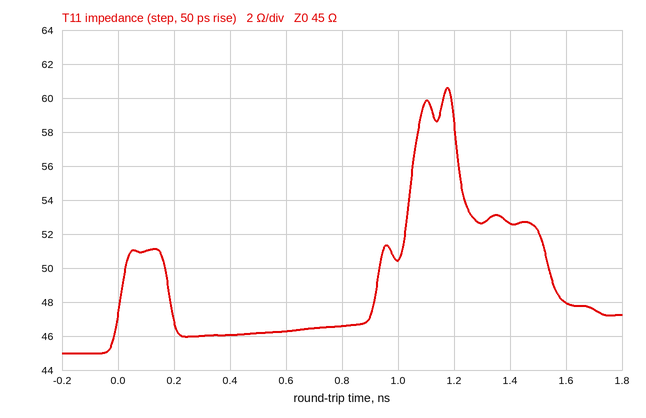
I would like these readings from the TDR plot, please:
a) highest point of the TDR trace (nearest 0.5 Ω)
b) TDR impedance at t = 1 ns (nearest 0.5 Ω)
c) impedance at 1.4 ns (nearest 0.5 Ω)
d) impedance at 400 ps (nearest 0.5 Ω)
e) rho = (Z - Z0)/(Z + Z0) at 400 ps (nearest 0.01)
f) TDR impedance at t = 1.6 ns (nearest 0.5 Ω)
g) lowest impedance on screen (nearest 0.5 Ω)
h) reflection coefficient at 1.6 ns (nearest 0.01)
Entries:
60.5 Ω
50.5 Ω
52.5 Ω
46.0 Ω
+0.01
48.0 Ω
45.0 Ω
+0.03
